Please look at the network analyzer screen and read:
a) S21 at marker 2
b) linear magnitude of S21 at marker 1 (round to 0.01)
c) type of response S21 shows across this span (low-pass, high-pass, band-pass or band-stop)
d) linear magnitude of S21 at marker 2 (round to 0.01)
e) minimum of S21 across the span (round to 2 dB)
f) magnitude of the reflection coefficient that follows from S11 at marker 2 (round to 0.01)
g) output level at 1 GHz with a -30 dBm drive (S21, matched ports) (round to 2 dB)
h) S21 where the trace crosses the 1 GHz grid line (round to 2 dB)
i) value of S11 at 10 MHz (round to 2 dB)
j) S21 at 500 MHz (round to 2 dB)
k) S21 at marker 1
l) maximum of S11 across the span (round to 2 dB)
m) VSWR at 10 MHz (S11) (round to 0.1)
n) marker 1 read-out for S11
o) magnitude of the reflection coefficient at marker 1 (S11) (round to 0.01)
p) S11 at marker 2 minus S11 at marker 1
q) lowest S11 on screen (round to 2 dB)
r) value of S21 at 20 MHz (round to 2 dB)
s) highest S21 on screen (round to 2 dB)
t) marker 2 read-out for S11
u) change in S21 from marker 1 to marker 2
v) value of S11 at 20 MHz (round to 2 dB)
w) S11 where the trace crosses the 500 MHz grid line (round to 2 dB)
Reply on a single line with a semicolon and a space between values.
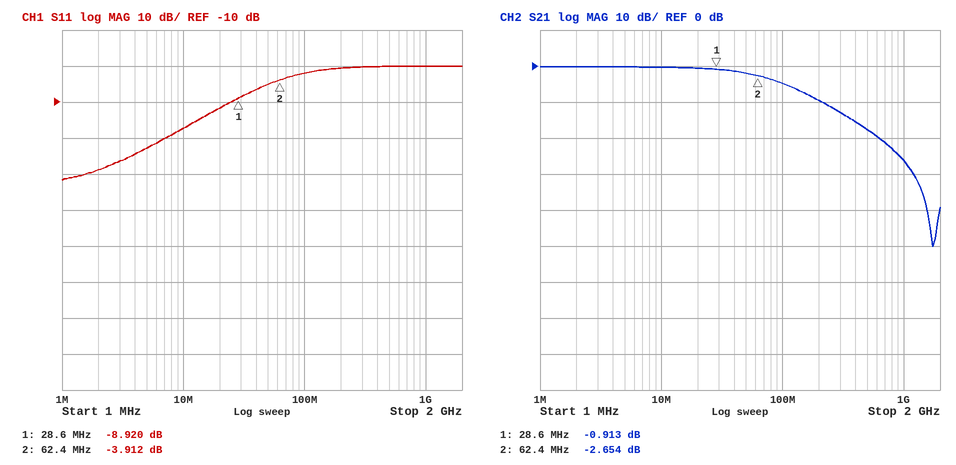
-2.654 dB; 0.90; low-pass; 0.74; -50 dB; 0.64; -56 dBm; -26 dB; -18 dB; -18 dB; -0.913 dB; 0 dB; 1.3; -8.920 dB; 0.36; 5.008 dB; -32 dB; 0 dB; 0 dB; -3.912 dB; -1.741 dB; -12 dB; 0 dB
